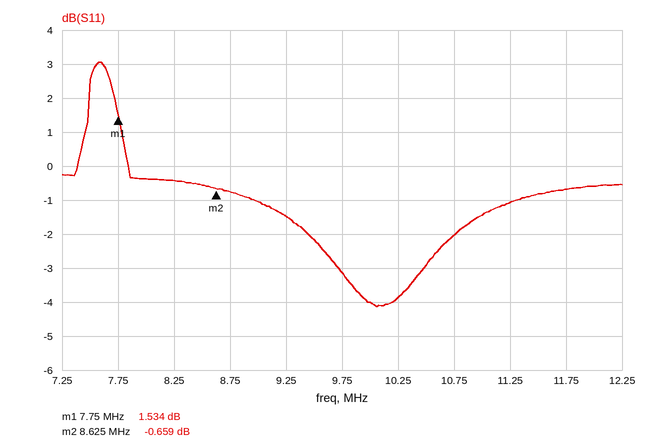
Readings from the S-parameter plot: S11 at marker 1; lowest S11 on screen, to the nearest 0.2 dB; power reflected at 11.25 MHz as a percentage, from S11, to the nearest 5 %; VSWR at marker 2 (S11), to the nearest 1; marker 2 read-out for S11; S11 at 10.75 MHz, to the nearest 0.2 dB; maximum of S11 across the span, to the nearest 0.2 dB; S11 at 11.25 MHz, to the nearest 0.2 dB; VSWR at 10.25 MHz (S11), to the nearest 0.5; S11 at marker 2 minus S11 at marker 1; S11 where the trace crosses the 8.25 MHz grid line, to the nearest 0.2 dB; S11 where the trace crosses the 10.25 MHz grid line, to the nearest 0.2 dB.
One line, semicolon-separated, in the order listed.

1.534 dB; -4.2 dB; 80 %; 26; -0.659 dB; -2.0 dB; 3.0 dB; -1.0 dB; 4.5; -2.193 dB; -0.4 dB; -3.8 dB
